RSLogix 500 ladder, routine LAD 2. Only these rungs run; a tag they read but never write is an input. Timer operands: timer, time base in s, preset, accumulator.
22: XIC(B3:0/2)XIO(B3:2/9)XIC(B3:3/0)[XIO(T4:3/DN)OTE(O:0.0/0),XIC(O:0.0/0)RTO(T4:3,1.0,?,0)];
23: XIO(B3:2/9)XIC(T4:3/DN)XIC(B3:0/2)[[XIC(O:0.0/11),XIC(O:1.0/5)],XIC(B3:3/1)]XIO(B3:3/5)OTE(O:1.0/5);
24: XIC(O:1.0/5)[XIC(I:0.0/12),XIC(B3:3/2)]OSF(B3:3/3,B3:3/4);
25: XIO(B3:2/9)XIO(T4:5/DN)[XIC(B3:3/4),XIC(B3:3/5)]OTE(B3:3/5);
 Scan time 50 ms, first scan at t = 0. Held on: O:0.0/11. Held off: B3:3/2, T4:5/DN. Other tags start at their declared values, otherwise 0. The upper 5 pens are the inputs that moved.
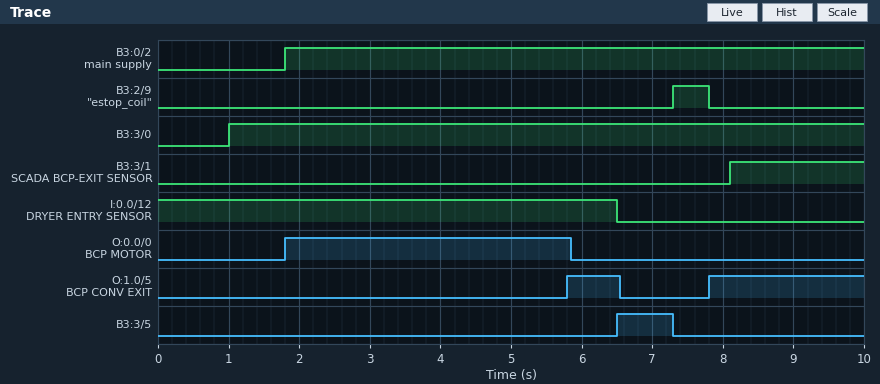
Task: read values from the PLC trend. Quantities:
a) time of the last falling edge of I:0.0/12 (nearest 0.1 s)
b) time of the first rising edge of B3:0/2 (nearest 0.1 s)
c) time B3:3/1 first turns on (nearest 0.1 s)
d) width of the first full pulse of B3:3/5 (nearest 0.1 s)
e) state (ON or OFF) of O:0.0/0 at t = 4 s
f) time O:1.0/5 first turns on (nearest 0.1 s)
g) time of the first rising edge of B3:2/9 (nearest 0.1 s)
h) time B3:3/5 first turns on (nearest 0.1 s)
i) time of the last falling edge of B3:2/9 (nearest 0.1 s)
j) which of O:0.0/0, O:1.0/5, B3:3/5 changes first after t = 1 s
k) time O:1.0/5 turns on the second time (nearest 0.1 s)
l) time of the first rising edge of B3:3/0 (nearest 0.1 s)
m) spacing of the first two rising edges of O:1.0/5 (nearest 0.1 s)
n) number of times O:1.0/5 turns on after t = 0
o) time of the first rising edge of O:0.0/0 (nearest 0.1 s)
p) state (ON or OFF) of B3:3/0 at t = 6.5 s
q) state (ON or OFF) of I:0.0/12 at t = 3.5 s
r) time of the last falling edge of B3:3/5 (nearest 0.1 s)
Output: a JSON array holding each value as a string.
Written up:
["6.5 s", "1.8 s", "8.1 s", "0.8 s", "ON", "5.8 s", "7.3 s", "6.5 s", "7.8 s", "O:0.0/0", "7.8 s", "1.0 s", "2.0 s", "2", "1.8 s", "ON", "ON", "7.3 s"]
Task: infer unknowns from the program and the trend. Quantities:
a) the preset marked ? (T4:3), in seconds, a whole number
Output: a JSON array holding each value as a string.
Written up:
["4 s"]
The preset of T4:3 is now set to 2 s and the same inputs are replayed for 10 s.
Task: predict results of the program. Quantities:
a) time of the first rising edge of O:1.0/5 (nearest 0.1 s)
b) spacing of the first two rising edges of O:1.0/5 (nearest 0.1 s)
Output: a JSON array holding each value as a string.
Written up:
["3.8 s", "4.0 s"]
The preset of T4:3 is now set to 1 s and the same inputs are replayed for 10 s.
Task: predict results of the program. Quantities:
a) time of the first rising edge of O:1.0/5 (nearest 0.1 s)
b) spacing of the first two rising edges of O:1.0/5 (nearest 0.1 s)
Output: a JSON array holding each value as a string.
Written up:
["2.8 s", "5.0 s"]
